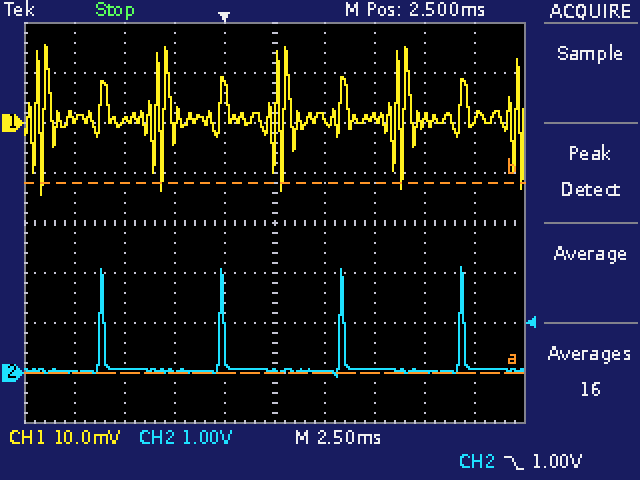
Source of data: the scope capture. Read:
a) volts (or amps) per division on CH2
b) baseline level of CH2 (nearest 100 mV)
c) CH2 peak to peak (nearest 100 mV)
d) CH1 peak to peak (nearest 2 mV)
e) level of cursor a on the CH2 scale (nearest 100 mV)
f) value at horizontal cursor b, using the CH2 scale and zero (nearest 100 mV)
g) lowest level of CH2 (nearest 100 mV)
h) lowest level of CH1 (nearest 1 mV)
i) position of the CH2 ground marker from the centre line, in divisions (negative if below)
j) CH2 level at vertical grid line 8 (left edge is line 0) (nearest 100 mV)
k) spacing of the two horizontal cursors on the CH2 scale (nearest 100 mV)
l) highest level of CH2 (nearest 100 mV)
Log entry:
1 V
100 mV
2.2 V
30 mV
0.0 V
3.8 V
-100 mV
-14 mV
-3.0 div
0.0 V
3.8 V
2.1 V
